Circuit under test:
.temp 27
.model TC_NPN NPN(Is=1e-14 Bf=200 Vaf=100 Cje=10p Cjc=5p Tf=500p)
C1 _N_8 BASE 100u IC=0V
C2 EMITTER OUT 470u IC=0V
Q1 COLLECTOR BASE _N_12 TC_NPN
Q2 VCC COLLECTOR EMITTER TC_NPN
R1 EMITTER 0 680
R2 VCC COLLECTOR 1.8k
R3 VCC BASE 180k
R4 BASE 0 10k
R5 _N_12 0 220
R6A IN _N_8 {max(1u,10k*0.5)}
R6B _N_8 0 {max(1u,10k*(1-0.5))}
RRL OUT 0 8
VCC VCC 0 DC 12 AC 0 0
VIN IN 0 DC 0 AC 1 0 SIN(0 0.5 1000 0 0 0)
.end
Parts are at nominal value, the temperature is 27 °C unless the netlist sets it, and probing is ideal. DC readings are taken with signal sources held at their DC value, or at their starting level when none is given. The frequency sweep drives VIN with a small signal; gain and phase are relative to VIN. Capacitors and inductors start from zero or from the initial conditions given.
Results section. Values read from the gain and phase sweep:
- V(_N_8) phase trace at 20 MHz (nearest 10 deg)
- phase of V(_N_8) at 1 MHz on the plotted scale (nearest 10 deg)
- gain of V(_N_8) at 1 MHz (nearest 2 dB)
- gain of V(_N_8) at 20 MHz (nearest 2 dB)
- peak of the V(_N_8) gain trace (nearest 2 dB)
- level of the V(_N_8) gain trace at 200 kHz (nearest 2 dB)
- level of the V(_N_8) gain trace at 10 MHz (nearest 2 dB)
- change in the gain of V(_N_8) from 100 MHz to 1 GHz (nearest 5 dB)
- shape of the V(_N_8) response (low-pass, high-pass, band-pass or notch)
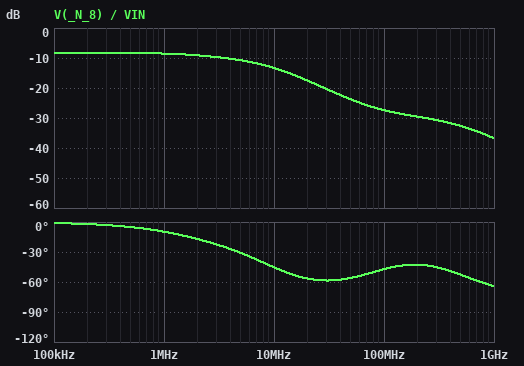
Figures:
-60 deg
-10 deg
-8 dB
-18 dB
-8 dB
-8 dB
-14 dB
-10 dB
low-pass
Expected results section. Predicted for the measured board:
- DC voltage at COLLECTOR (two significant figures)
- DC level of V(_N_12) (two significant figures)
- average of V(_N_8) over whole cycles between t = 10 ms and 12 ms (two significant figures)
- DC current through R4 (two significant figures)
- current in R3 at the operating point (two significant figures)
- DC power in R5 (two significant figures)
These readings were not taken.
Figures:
12 V
28 mV
130 mV
63 µA
63 µA
3.5 µW
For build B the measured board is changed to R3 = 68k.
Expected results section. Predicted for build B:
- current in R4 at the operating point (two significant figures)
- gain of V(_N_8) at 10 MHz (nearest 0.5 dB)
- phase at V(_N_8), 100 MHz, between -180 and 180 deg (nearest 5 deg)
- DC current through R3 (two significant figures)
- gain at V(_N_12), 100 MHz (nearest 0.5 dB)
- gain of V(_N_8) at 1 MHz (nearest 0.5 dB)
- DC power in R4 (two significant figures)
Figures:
140 µA
-12.5 dB
-65 deg
160 µA
-24.5 dB
-9.0 dB
200 µW
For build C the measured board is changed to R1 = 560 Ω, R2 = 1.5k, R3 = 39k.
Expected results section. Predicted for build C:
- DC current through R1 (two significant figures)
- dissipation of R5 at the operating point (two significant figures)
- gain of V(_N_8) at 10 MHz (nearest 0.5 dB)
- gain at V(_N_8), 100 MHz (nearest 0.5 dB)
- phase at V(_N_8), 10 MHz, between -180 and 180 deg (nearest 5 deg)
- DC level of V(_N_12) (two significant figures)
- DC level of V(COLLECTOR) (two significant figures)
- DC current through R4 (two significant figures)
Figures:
2.3 mA
9.9 mW
-16.0 dB
-27.5 dB
-30 deg
1.5 V
2.0 V
220 µA
